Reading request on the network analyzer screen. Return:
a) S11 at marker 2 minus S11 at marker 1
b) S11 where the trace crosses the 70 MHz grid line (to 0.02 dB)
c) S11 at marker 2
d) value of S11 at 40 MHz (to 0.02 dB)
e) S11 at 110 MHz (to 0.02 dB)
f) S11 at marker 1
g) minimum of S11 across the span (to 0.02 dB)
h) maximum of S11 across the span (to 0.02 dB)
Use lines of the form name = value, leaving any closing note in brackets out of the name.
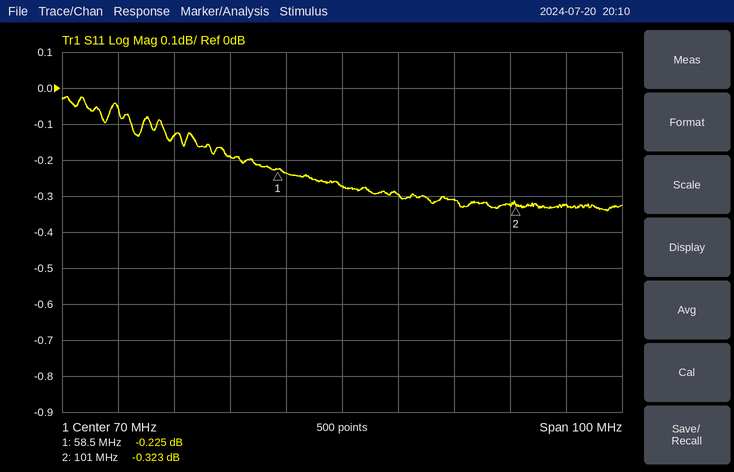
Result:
S11 at marker 2 minus S11 at marker 1 = -0.098 dB
S11 where the trace crosses the 70 MHz grid line = -0.28 dB
S11 at marker 2 = -0.323 dB
value of S11 at 40 MHz = -0.14 dB
S11 at 110 MHz = -0.32 dB
S11 at marker 1 = -0.225 dB
minimum of S11 across the span = -0.34 dB
maximum of S11 across the span = -0.02 dB
